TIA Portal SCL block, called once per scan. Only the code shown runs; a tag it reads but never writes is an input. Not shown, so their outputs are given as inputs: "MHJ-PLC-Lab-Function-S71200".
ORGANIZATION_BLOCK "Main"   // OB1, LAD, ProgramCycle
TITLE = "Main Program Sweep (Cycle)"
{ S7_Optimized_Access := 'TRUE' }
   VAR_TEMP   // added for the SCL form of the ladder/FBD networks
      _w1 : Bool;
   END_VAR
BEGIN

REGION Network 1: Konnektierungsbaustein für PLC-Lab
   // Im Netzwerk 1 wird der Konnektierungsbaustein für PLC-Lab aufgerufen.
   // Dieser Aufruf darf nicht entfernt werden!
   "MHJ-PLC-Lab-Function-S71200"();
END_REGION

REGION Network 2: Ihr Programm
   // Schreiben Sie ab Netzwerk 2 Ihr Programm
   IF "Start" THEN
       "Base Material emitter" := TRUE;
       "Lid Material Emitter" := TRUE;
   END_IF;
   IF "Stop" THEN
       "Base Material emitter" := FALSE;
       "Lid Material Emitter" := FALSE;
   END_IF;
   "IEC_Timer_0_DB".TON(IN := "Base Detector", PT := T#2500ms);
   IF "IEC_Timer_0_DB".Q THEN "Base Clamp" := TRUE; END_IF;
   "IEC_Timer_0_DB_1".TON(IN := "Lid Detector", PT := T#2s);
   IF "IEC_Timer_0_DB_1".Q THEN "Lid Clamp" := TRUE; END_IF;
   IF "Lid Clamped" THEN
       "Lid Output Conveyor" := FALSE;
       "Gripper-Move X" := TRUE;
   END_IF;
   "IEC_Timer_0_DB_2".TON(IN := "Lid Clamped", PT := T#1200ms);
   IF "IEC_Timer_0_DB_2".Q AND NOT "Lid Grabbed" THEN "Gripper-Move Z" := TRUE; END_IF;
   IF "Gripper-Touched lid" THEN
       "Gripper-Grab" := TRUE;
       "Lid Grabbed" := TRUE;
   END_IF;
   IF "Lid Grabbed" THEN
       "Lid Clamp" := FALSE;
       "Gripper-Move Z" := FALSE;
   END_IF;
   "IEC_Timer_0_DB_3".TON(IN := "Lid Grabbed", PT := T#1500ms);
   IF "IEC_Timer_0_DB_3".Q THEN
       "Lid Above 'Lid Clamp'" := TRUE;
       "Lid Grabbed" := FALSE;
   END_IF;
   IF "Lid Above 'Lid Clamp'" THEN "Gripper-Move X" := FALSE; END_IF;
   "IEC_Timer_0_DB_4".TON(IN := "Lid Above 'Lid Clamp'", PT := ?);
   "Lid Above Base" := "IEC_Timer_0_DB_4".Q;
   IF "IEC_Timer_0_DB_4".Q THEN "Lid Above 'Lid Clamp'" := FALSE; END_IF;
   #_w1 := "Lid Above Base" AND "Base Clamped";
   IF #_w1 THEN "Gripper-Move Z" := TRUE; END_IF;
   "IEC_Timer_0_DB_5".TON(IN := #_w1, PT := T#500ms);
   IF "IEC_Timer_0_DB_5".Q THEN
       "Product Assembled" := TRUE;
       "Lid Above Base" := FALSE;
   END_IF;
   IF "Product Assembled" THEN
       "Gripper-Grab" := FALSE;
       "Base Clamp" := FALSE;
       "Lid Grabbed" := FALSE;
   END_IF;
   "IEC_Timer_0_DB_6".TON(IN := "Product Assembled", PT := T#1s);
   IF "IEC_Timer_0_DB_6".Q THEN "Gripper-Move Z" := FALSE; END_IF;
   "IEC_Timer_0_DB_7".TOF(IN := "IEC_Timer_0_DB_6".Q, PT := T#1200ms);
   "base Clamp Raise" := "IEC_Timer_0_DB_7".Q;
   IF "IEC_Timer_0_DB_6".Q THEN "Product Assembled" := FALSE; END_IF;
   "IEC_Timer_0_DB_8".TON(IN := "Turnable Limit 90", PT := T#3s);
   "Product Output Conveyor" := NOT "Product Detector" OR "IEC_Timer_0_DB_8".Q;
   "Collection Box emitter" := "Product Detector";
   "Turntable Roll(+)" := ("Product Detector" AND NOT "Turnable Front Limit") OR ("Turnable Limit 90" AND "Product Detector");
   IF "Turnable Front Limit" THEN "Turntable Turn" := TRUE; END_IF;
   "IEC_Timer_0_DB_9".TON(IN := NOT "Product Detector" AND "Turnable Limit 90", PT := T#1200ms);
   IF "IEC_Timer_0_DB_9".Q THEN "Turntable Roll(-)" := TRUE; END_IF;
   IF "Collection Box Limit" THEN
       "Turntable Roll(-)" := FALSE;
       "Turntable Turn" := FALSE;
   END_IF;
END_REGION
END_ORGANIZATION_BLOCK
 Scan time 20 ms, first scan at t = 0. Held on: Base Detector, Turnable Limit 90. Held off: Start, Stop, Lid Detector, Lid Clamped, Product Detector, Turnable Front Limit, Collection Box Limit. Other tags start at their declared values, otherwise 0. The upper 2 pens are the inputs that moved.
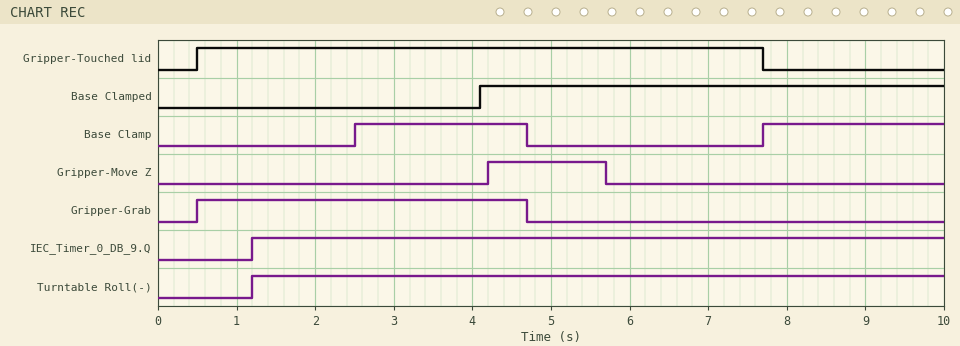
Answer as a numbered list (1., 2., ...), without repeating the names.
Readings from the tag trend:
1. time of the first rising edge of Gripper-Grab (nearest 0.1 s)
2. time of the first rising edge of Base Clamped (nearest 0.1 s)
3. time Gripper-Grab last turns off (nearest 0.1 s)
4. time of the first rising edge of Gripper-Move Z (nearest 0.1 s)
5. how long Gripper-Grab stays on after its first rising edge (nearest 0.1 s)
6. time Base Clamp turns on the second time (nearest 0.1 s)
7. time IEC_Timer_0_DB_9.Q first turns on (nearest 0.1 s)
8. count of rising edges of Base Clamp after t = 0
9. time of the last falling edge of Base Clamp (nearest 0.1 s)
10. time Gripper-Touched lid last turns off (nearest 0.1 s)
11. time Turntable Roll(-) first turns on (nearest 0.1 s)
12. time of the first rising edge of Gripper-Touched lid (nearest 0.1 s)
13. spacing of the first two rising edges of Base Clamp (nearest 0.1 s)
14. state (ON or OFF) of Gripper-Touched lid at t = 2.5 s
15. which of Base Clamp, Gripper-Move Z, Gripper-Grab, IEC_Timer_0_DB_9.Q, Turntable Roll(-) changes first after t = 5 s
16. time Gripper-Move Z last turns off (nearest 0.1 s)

1. 0.5 s
2. 4.1 s
3. 4.7 s
4. 4.2 s
5. 4.2 s
6. 7.7 s
7. 1.2 s
8. 2
9. 4.7 s
10. 7.7 s
11. 1.2 s
12. 0.5 s
13. 5.2 s
14. ON
15. Gripper-Move Z
16. 5.7 s
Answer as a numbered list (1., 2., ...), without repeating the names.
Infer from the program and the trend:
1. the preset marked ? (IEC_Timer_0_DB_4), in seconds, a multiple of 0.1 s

1. 2.2 s
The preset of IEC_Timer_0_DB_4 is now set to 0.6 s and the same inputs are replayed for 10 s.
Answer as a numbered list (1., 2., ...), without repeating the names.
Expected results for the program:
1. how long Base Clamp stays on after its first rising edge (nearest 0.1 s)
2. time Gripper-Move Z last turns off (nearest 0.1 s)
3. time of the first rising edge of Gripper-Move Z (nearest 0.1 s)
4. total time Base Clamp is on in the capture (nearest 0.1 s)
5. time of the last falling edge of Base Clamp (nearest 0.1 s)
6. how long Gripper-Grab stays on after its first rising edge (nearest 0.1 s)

1. 2.1 s
2. 5.6 s
3. 4.1 s
4. 4.4 s
5. 4.6 s
6. 4.1 s
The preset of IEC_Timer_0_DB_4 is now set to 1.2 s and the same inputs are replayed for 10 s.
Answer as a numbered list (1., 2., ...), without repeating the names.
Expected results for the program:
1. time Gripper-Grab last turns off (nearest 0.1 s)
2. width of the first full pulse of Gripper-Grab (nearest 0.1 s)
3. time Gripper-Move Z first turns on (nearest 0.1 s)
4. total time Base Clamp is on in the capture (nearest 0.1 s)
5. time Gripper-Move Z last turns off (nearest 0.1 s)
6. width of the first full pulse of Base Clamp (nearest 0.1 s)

1. 4.6 s
2. 4.1 s
3. 4.1 s
4. 4.4 s
5. 5.6 s
6. 2.1 s
